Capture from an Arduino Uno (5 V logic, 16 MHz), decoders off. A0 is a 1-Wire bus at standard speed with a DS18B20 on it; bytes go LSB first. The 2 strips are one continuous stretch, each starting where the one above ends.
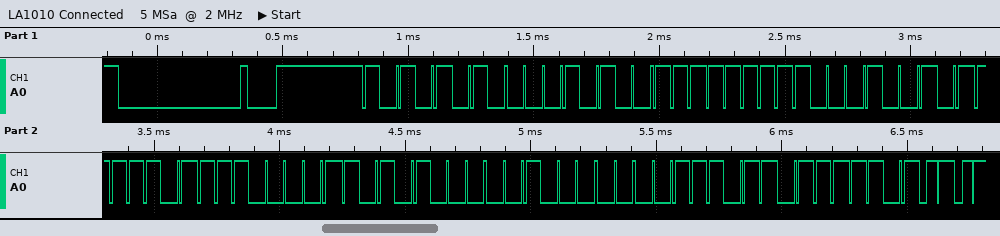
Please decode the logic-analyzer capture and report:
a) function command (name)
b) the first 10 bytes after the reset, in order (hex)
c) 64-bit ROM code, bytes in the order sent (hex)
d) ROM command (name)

Read Scratchpad
55 28 FF 91 BE 87 15 04 DC BE
28 FF 91 BE 87 15 04 DC
Match ROM
